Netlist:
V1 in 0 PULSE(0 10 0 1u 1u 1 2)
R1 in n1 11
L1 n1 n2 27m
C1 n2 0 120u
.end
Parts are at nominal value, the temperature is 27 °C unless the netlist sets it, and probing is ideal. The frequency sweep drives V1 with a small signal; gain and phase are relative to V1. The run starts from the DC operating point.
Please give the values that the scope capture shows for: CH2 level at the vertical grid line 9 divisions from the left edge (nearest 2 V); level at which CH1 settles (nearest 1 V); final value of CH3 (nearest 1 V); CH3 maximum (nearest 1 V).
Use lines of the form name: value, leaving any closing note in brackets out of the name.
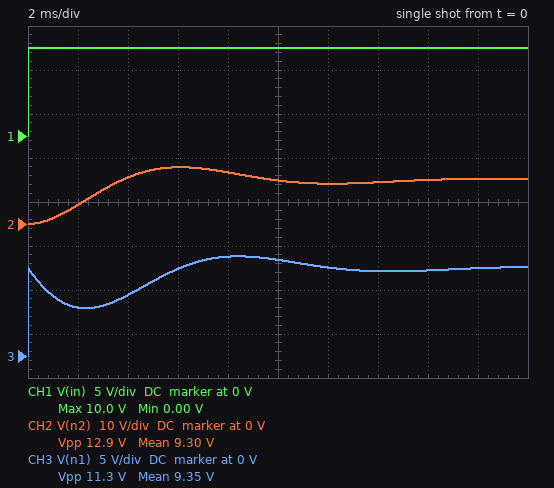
CH2 level at the vertical grid line 9 divisions from the left edge: 10 V
level at which CH1 settles: 10 V
final value of CH3: 10 V
CH3 maximum: 11 V
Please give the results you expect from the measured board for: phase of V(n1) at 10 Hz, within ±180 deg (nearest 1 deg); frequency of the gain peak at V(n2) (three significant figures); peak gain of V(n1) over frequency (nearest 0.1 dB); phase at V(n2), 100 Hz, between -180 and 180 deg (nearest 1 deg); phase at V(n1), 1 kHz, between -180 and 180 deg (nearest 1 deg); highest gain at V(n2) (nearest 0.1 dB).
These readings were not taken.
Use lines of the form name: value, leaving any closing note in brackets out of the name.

phase of V(n1) at 10 Hz, within ±180 deg: -5 deg
frequency of the gain peak at V(n2): 75.6 Hz
peak gain of V(n1) over frequency: 0 dB
phase at V(n2), 100 Hz, between -180 and 180 deg: -109 deg
phase at V(n1), 1 kHz, between -180 and 180 deg: 4 deg
highest gain at V(n2): 3.3 dB
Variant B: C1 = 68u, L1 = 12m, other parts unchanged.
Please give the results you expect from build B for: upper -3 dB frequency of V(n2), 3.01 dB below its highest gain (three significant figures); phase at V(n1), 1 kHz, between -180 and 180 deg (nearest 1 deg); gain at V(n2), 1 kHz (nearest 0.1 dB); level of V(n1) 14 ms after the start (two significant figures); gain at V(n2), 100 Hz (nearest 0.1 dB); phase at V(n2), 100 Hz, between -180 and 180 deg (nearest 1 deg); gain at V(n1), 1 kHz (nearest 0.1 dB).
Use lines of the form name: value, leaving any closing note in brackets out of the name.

upper -3 dB frequency of V(n2), 3.01 dB below its highest gain: 209 Hz
phase at V(n1), 1 kHz, between -180 and 180 deg: 9 deg
gain at V(n2), 1 kHz: -30.0 dB
level of V(n1) 14 ms after the start: 10 V
gain at V(n2), 100 Hz: 1.7 dB
phase at V(n2), 100 Hz, between -180 and 180 deg: -35 deg
gain at V(n1), 1 kHz: -0.1 dB
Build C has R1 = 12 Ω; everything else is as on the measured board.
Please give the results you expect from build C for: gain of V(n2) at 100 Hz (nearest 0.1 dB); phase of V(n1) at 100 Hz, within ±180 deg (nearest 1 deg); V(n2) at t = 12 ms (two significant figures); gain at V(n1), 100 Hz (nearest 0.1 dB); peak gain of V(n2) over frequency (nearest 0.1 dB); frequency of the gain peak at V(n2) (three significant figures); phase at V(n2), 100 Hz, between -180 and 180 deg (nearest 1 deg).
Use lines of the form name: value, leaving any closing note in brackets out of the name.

gain of V(n2) at 100 Hz: 0.5 dB
phase of V(n1) at 100 Hz, within ±180 deg: 73 deg
V(n2) at t = 12 ms: 9.4 V
gain at V(n1), 100 Hz: -10.6 dB
peak gain of V(n2) over frequency: 2.7 dB
frequency of the gain peak at V(n2): 72.9 Hz
phase at V(n2), 100 Hz, between -180 and 180 deg: -107 deg
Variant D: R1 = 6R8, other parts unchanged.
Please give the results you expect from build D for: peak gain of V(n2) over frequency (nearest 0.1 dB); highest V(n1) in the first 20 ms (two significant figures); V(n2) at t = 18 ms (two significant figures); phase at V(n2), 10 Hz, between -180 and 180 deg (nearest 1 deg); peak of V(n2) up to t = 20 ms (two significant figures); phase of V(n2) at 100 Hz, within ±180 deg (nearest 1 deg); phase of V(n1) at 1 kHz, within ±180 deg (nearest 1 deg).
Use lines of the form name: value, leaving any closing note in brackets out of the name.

peak gain of V(n2) over frequency: 7.1 dB
highest V(n1) in the first 20 ms: 12 V
V(n2) at t = 18 ms: 11 V
phase at V(n2), 10 Hz, between -180 and 180 deg: -3 deg
peak of V(n2) up to t = 20 ms: 15 V
phase of V(n2) at 100 Hz, within ±180 deg: -119 deg
phase of V(n1) at 1 kHz, within ±180 deg: 2 deg
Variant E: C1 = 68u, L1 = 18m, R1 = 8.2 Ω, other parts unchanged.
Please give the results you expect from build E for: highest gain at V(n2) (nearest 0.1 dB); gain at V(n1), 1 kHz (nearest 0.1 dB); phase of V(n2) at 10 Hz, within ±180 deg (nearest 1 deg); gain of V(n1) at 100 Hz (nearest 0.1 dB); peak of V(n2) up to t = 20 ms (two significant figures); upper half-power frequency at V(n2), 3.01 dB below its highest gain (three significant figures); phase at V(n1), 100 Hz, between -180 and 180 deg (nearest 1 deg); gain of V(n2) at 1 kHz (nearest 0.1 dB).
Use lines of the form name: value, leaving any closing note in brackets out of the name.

highest gain at V(n2): 6.2 dB
gain at V(n1), 1 kHz: 0 dB
phase of V(n2) at 10 Hz, within ±180 deg: -2 deg
gain of V(n1) at 100 Hz: -1.6 dB
peak of V(n2) up to t = 20 ms: 14 V
upper half-power frequency at V(n2), 3.01 dB below its highest gain: 168 Hz
phase at V(n1), 100 Hz, between -180 and 180 deg: -34 deg
gain of V(n2) at 1 kHz: -33.5 dB
